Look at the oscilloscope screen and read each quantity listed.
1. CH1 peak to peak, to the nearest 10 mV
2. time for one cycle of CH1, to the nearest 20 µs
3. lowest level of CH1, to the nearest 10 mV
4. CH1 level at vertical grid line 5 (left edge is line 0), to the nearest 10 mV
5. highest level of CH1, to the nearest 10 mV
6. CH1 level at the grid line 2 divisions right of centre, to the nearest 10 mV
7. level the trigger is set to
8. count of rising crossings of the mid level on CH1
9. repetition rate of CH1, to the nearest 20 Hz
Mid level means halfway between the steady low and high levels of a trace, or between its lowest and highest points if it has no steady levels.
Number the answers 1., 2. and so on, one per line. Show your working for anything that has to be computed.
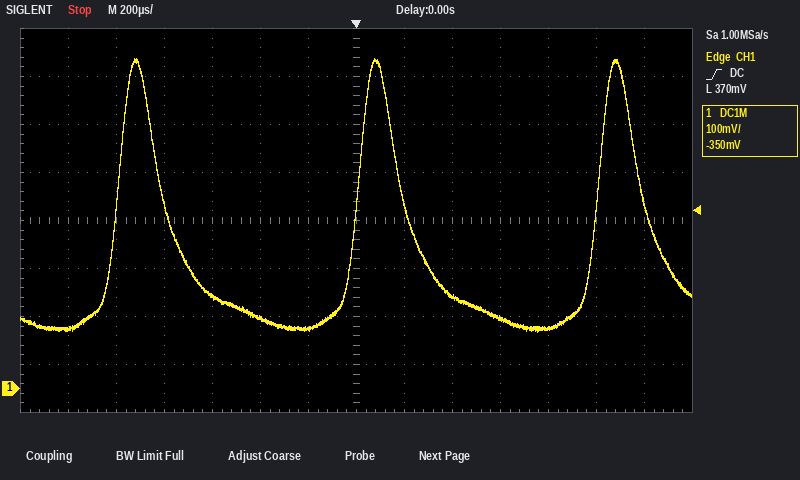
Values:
1. 690 mV − (120 mV) = 570 mV
2. 1.00 ms
3. 120 mV
4. 150 mV
5. 690 mV
6. 190 mV
7. 370 mV
8. 3
9. 1 / 1.00 ms ≈ 1.00 kHz
